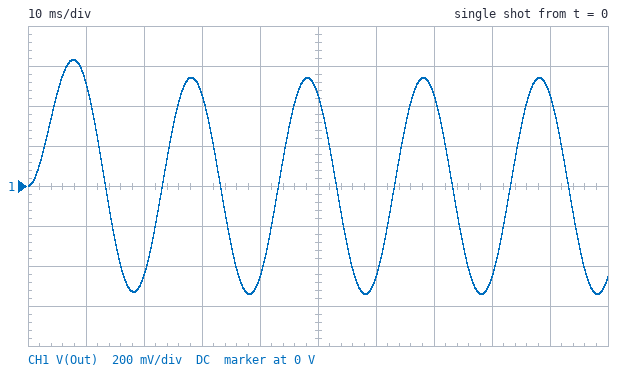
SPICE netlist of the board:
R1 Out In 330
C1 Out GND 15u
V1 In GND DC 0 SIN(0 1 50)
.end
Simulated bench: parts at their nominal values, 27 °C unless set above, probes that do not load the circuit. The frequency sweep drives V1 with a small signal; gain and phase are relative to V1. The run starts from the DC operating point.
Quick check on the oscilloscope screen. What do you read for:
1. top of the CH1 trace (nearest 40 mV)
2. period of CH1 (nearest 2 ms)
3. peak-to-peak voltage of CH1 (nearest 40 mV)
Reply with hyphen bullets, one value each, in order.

- 640 mV
- 20 ms
- 1.16 V
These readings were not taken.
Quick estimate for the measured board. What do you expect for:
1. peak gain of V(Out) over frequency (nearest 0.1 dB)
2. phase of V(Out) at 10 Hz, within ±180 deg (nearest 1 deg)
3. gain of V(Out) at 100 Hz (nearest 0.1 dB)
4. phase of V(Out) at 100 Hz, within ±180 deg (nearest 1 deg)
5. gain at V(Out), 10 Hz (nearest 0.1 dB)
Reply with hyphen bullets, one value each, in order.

- 0 dB
- -17 deg
- -10.3 dB
- -72 deg
- -0.4 dB
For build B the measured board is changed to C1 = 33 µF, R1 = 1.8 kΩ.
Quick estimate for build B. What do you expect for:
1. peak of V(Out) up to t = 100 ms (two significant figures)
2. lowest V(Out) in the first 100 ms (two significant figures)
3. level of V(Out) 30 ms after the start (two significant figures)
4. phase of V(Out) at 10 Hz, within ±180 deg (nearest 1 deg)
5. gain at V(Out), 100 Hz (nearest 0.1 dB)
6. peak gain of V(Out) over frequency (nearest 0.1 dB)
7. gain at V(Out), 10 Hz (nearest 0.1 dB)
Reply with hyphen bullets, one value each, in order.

- 99 mV
- -44 mV
- 86 mV
- -75 deg
- -31.4 dB
- 0 dB
- -11.7 dB
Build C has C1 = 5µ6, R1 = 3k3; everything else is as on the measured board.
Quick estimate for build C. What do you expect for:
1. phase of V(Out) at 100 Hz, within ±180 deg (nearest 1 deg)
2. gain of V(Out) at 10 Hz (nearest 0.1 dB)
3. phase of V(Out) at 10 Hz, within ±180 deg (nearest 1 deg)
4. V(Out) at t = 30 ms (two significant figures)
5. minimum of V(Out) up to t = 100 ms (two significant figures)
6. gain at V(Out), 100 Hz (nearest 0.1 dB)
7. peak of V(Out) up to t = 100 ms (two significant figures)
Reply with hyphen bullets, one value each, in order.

- -85 deg
- -3.7 dB
- -49 deg
- 200 mV
- -170 mV
- -21.3 dB
- 270 mV
